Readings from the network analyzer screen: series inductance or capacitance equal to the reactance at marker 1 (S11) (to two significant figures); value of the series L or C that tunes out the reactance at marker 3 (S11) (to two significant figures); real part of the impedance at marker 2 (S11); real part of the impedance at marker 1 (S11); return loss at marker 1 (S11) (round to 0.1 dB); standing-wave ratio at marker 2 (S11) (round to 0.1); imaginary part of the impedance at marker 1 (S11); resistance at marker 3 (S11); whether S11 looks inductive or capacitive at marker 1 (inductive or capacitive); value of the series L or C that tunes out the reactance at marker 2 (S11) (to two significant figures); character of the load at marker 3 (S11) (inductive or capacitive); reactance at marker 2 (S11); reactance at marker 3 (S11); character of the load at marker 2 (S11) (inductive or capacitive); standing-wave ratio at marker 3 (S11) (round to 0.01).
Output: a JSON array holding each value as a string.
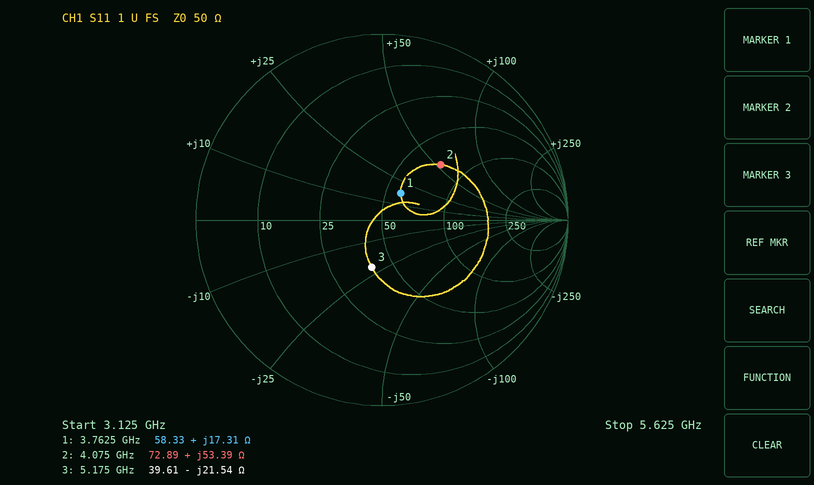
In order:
["730 pH", "660 pH", "72.89 Ω", "58.33 Ω", "15.1 dB", "2.5", "+17.31 Ω", "39.61 Ω", "inductive", "730 fF", "capacitive", "+53.39 Ω", "-21.54 Ω", "inductive", "1.70"]
